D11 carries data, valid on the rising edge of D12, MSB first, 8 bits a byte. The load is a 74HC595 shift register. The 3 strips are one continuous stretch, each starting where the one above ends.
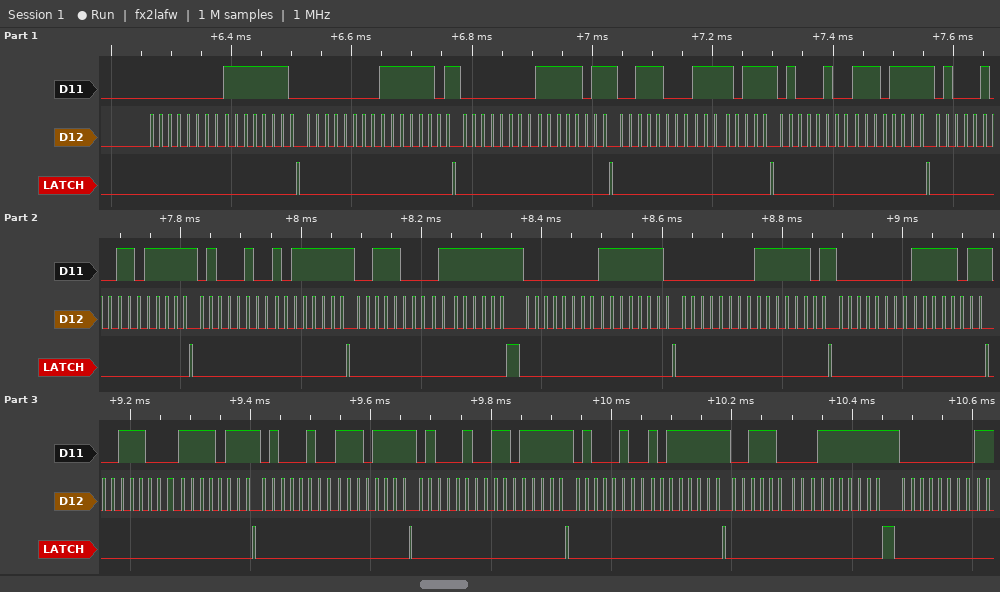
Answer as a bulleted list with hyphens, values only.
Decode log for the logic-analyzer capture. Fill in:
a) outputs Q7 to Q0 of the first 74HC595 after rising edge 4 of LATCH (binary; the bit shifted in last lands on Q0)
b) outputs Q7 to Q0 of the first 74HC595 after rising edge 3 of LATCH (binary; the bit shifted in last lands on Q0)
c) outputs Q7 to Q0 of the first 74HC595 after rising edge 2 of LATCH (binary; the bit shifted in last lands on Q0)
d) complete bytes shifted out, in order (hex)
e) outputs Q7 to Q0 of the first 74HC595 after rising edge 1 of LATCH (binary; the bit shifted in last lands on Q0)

- 11110111
- 11111011
- 11111101
- 00 FE 00 FD 00 FB 38 F7 44 EF 44 DF 44 BF 38 7F 00 FE 00 FD 00 FB 38 F7 44 EF 44 DF 44 BF 38 7F 00
- 11111110
